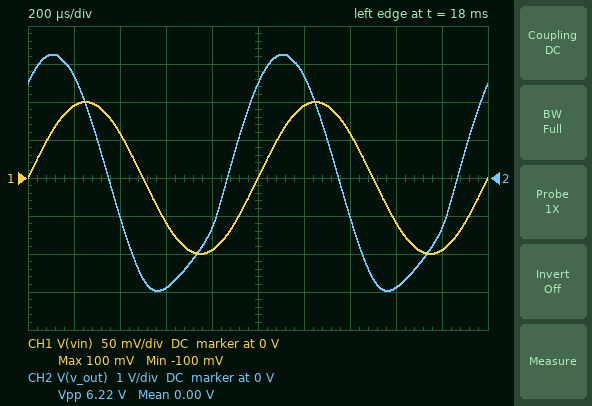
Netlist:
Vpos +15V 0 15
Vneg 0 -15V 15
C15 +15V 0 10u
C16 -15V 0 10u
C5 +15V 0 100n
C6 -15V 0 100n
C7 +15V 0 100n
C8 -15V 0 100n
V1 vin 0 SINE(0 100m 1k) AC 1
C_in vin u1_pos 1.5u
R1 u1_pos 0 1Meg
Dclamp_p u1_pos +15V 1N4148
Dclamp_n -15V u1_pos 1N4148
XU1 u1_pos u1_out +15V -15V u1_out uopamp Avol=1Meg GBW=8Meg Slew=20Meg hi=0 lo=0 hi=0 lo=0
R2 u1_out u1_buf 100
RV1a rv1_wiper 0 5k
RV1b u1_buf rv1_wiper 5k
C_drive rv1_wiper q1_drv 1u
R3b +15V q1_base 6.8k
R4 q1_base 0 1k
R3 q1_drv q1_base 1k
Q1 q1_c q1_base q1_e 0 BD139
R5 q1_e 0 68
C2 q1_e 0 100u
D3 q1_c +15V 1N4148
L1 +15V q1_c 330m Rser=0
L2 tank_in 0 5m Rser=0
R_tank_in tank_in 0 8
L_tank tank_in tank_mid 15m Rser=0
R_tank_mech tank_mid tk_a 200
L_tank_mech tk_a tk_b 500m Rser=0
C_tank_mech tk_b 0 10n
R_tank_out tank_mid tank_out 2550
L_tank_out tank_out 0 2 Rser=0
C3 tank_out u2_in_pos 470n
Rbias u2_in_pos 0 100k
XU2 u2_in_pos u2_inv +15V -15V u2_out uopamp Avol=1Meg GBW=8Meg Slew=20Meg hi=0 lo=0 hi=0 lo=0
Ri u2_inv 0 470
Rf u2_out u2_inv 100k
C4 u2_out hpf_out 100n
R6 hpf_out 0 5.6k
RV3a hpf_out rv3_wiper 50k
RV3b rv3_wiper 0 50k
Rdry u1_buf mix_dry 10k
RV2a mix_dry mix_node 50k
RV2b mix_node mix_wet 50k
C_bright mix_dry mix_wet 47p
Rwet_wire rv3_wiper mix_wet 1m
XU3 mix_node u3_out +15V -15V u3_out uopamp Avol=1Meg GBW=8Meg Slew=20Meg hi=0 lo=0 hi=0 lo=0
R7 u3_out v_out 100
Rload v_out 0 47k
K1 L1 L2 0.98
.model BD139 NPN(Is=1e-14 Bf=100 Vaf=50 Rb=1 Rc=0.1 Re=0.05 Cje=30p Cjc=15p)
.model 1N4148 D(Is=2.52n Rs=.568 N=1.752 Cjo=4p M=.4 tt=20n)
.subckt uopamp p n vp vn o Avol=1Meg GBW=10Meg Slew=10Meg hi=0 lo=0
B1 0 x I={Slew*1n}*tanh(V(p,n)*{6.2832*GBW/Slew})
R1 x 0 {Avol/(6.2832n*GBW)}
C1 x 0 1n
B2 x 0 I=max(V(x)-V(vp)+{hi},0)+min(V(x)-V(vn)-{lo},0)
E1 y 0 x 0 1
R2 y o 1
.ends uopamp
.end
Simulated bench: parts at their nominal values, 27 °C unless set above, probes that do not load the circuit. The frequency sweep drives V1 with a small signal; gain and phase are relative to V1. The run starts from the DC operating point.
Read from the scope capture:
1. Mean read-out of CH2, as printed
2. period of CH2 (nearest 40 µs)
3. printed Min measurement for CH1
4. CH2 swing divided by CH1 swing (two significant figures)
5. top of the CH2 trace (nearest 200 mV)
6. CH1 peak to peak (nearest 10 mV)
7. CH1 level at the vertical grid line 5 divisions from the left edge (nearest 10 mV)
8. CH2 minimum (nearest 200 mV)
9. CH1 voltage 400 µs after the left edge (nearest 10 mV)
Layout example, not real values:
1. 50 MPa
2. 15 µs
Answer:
1. 0.00 V
2. 1.00 ms
3. -100 mV
4. 31
5. 3.2 V
6. 200 mV
7. 0 V
8. -3.0 V
9. 60 mV
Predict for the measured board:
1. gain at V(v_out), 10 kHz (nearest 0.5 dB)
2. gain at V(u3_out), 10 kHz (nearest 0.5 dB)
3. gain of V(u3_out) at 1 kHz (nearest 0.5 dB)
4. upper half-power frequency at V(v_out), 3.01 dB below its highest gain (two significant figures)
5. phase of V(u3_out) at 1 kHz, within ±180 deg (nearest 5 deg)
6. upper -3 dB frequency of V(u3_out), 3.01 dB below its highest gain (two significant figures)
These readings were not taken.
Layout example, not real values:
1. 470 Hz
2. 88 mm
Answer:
1. 31.0 dB
2. 31.0 dB
3. 30.5 dB
4. 2.2 kHz
5. 55 deg
6. 2.2 kHz
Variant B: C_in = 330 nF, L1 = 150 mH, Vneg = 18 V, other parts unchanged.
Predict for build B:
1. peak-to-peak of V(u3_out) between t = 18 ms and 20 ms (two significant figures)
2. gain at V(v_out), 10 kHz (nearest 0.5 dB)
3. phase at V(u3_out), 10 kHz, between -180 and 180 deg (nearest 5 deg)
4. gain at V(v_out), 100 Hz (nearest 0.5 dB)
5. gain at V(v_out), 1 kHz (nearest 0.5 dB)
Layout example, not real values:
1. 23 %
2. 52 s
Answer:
1. 4.7 V
2. 28.0 dB
3. -15 deg
4. -2.0 dB
5. 27.5 dB
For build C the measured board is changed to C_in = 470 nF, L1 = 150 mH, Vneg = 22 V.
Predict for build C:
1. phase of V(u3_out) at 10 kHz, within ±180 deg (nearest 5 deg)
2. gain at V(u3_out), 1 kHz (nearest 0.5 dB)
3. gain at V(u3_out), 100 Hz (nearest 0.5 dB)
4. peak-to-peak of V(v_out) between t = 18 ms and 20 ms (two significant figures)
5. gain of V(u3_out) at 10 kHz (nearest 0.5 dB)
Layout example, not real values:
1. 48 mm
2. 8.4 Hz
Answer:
1. -15 deg
2. 27.5 dB
3. -2.0 dB
4. 4.7 V
5. 28.0 dB
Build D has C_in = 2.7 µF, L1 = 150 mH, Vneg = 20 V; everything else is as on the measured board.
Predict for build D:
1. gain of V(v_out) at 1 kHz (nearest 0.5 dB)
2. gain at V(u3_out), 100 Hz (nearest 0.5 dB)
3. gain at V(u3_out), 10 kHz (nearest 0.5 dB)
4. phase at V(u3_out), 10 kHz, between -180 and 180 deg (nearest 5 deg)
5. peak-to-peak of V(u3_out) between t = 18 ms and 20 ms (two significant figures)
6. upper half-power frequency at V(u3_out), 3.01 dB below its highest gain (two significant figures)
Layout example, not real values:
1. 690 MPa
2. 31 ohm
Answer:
1. 27.5 dB
2. -2.0 dB
3. 28.0 dB
4. -15 deg
5. 4.7 V
6. 2.2 kHz
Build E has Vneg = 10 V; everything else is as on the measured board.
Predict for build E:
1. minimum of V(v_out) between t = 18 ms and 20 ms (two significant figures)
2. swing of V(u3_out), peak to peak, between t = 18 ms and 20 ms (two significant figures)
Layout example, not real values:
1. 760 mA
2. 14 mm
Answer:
1. -2.8 V
2. 5.9 V
